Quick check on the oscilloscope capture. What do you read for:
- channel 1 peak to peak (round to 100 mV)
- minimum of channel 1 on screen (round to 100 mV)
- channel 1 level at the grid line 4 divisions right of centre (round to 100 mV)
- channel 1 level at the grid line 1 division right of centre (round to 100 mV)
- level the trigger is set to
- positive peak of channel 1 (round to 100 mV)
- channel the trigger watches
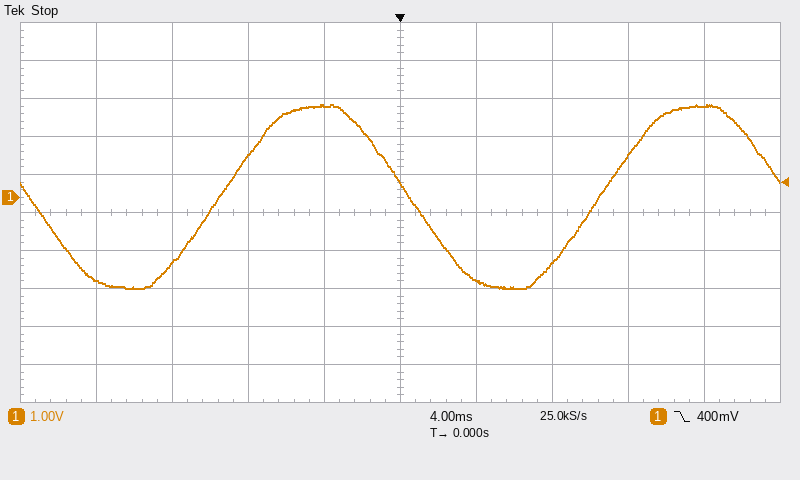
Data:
4.8 V
-2.4 V
2.4 V
-2.2 V
400 mV
2.4 V
channel 1
